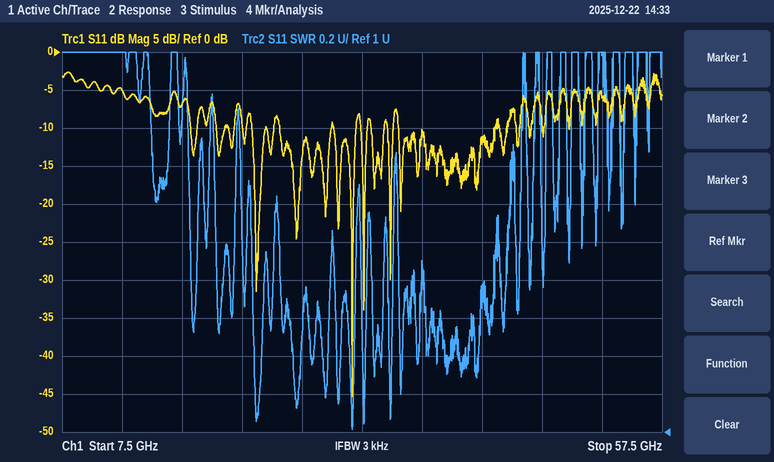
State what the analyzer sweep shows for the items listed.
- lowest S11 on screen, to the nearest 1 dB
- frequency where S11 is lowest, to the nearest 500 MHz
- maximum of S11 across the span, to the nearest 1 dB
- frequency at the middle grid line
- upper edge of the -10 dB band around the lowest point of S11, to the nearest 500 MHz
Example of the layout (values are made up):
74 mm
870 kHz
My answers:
-45 dB
31.5 GHz
-3 dB
32.5 GHz
32.0 GHz
